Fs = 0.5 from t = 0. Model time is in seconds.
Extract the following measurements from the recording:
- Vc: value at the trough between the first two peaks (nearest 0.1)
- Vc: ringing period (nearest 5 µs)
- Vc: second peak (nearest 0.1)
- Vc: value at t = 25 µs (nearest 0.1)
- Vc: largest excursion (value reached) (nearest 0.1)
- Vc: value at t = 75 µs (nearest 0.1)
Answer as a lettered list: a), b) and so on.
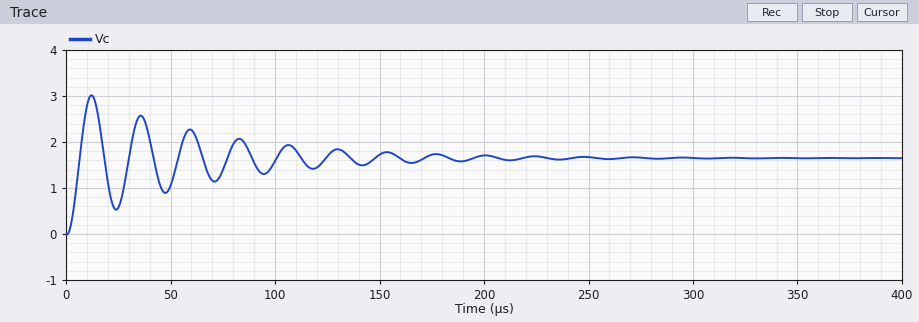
a) 0.5
b) 25 µs
c) 2.6
d) 0.6
e) 3.0
f) 1.4
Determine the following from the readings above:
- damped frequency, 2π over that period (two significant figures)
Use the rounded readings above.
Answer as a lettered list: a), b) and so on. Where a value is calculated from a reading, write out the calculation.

a) 2π / 25 = 0.25 rad/µs
